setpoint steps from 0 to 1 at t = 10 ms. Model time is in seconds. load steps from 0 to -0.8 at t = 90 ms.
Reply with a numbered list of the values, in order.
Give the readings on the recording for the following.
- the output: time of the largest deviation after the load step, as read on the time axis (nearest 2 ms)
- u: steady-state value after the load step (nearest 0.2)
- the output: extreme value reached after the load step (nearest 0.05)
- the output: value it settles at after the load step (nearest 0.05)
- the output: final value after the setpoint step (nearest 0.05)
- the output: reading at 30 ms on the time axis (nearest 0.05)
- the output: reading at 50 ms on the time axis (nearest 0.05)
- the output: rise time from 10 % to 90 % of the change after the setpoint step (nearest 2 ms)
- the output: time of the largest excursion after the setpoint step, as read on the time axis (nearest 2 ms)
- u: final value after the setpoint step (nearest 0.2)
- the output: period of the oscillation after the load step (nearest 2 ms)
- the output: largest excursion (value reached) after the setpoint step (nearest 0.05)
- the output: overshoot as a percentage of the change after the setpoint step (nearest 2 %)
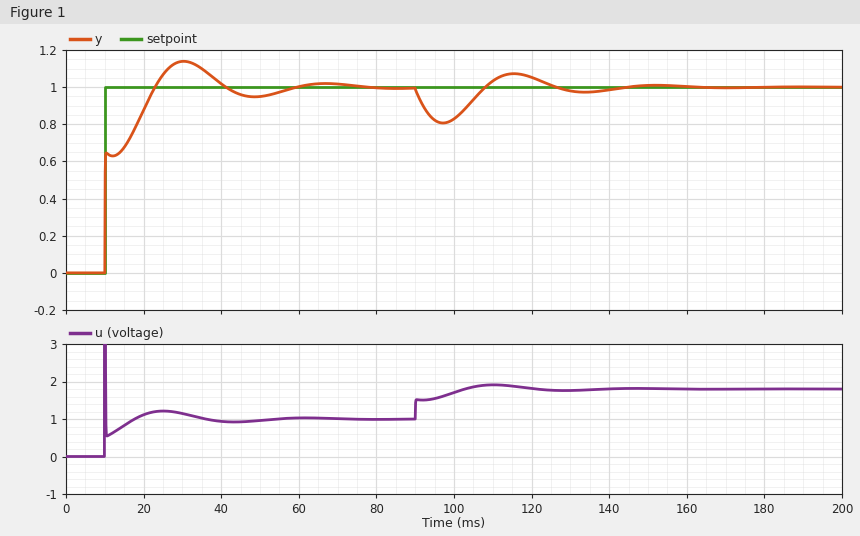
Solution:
1. 98 ms
2. 1.8
3. 0.80
4. 1.00
5. 1.00
6. 1.15
7. 0.95
8. 10 ms
9. 30 ms
10. 1.0
11. 36 ms
12. 1.15
13. 14 %
